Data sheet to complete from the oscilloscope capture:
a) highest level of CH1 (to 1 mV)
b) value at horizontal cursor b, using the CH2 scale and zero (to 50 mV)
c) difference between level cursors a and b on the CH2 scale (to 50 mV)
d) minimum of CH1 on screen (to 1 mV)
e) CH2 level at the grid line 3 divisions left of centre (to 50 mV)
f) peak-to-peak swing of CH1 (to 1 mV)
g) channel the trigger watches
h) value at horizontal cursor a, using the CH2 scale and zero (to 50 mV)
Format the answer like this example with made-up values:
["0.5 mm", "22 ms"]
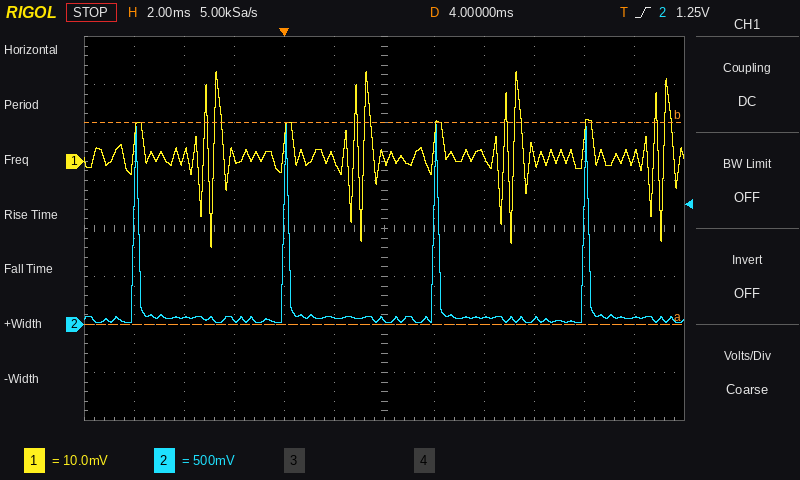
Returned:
["19 mV", "2.10 V", "2.10 V", "-18 mV", "50 mV", "37 mV", "CH2", "0 mV"]
